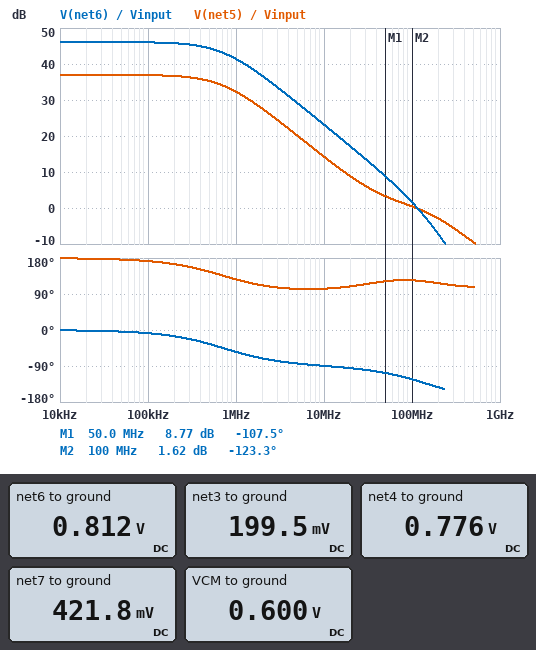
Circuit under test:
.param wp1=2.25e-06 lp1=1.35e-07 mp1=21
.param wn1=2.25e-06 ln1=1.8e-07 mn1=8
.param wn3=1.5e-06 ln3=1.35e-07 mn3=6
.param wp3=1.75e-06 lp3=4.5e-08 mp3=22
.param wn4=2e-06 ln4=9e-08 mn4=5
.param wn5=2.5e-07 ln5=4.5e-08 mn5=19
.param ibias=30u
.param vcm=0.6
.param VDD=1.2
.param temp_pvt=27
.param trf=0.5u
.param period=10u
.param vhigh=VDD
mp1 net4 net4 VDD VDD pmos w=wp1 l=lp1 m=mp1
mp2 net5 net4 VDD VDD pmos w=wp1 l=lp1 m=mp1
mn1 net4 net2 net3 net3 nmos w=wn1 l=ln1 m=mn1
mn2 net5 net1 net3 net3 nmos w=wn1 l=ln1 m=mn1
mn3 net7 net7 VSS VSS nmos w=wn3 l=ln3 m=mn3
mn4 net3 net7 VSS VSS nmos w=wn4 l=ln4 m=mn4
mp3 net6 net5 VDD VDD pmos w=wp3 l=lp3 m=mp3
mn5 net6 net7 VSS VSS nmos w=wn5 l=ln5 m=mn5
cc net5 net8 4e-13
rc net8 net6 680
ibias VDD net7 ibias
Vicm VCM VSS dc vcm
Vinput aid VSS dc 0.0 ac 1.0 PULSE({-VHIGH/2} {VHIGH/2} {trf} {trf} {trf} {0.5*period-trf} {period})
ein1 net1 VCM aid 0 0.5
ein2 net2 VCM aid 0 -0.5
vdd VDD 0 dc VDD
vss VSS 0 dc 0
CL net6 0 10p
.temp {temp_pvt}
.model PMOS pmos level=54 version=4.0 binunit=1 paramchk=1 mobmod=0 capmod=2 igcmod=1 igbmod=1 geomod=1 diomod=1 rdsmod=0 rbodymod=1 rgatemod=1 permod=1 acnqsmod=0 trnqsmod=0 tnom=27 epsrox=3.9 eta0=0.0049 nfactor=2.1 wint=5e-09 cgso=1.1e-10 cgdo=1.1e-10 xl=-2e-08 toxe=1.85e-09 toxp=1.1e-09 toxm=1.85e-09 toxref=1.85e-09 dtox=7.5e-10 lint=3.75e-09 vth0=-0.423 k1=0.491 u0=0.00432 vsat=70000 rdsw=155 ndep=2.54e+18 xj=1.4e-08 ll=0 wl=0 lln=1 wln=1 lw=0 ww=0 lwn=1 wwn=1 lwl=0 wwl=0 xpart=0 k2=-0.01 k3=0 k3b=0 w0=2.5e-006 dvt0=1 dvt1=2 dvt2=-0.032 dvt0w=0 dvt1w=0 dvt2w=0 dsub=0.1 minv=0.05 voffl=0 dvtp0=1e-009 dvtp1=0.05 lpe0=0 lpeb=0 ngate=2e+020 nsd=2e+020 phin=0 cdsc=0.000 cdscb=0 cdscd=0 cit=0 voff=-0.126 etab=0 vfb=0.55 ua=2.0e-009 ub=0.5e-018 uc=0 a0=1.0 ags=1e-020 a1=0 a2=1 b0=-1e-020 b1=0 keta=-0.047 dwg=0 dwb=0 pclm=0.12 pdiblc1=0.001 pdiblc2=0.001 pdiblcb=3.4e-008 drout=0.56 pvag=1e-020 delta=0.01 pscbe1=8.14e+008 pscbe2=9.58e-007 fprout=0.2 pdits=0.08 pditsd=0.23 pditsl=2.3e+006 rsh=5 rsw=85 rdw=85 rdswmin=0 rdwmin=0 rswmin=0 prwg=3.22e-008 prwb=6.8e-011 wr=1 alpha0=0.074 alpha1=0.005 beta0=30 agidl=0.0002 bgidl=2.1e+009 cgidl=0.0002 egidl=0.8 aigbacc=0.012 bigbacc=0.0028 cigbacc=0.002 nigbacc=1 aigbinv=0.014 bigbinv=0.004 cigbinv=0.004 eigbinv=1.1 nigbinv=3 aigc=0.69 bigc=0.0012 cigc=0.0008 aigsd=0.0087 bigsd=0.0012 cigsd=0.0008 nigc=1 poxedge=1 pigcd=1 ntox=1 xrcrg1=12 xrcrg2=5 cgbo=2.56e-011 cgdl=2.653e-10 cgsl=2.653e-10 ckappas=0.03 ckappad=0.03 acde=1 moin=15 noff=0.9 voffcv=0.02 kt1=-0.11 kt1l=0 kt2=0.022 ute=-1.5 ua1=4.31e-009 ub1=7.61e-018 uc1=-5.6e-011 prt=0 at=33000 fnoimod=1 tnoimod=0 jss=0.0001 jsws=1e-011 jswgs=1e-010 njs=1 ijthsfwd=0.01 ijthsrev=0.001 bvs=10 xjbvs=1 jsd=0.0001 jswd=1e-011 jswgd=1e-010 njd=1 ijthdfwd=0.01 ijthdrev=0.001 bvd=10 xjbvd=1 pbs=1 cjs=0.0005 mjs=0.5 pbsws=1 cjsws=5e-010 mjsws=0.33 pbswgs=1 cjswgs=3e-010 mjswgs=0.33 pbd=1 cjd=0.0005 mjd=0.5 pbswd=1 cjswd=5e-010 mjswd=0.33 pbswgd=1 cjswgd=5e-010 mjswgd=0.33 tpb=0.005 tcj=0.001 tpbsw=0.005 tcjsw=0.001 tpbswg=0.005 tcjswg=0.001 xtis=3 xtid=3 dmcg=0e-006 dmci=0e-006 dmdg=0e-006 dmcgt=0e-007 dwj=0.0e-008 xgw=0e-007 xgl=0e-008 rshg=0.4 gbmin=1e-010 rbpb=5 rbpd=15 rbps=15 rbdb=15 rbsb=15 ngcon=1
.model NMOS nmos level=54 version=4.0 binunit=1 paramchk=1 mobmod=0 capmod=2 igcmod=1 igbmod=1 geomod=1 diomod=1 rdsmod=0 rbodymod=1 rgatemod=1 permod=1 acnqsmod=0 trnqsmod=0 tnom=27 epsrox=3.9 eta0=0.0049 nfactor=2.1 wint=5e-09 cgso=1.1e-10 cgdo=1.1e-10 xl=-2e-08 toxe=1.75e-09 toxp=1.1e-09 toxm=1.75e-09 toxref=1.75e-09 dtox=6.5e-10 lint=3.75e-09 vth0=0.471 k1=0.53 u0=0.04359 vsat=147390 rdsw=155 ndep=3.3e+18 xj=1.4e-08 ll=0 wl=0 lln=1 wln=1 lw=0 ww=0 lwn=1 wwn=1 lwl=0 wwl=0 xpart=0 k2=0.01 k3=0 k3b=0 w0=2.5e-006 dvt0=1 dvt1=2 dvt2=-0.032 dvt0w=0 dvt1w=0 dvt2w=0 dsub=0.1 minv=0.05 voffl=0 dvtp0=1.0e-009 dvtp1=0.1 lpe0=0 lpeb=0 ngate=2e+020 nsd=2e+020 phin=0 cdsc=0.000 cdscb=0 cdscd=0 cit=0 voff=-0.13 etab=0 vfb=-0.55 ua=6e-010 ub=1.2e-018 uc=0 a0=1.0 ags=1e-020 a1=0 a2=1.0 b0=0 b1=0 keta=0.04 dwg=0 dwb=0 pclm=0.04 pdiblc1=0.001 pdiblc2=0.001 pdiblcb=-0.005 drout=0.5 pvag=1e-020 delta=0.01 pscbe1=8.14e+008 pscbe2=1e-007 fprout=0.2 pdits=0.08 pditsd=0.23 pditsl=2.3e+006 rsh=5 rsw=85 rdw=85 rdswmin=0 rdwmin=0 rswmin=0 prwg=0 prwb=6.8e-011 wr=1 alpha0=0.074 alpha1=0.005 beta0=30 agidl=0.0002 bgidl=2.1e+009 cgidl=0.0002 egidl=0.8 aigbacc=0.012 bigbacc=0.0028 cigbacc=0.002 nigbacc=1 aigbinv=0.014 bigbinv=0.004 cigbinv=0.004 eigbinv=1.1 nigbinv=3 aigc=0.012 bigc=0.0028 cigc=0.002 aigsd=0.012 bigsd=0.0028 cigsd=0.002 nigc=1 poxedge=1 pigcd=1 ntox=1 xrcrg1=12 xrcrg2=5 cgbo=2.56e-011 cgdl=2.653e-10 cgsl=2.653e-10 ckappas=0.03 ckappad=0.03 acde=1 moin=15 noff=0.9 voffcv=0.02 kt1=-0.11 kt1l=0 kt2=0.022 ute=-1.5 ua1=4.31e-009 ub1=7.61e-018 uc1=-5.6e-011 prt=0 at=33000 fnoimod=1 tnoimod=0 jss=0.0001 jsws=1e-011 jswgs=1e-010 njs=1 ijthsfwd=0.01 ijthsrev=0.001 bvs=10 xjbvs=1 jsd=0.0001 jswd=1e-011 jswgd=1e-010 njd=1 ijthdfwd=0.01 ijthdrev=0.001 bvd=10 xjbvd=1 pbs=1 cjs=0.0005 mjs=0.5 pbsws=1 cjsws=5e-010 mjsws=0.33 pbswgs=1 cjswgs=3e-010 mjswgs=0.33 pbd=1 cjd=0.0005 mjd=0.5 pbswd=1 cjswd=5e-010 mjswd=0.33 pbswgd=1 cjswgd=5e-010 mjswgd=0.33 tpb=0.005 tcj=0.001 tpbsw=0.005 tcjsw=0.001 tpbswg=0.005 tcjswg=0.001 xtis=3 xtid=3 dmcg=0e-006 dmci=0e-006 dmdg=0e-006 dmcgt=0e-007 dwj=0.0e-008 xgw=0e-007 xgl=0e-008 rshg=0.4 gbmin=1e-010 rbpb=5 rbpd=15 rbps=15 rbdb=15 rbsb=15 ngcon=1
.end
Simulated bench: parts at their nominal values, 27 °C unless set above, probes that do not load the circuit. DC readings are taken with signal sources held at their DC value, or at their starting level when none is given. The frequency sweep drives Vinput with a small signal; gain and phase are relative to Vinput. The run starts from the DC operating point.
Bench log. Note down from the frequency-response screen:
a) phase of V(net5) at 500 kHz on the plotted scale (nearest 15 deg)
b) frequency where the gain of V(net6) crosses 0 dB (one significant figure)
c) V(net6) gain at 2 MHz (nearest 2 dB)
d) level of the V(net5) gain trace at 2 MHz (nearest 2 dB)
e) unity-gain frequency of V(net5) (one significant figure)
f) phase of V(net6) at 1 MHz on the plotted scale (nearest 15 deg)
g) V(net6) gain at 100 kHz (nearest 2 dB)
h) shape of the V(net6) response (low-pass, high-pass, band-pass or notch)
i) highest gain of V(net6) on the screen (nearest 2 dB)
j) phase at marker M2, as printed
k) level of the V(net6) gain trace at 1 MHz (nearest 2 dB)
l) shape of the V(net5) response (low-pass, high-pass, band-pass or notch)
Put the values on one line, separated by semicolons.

150 deg; 100 MHz; 36 dB; 28 dB; 100 MHz; -60 deg; 46 dB; low-pass; 46 dB; -123.3 deg; 42 dB; low-pass
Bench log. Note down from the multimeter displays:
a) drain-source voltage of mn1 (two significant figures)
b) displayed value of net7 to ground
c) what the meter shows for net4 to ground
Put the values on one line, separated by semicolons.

580 mV; 421.8 mV; 0.776 V
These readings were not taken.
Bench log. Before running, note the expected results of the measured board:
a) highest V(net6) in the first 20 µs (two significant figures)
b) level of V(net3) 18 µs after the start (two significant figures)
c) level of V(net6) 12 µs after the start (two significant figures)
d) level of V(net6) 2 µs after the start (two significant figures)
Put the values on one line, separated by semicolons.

1.2 V; 460 mV; 1.2 V; 1.2 V
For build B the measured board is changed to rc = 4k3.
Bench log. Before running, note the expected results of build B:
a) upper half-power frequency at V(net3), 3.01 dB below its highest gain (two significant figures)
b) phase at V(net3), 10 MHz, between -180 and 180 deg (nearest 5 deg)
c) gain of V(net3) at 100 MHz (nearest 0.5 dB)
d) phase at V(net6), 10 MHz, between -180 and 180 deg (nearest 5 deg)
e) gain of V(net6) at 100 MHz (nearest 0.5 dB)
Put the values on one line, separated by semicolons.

710 kHz; 120 deg; -43.0 dB; -85 deg; 5.0 dB
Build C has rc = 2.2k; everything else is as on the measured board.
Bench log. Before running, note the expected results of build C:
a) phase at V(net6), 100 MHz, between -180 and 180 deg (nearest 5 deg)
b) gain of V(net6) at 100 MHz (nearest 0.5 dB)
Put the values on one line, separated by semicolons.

-105 deg; 2.5 dB
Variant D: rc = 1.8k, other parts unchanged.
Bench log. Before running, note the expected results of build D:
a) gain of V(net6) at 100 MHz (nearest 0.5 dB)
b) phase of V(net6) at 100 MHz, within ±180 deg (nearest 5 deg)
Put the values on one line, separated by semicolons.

2.5 dB; -110 deg
